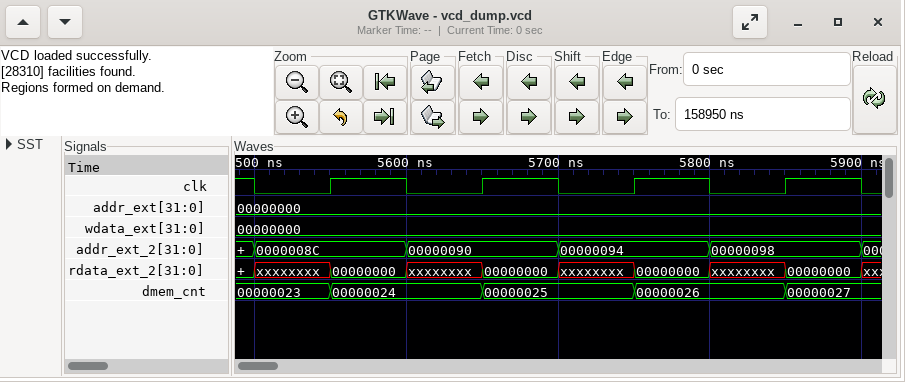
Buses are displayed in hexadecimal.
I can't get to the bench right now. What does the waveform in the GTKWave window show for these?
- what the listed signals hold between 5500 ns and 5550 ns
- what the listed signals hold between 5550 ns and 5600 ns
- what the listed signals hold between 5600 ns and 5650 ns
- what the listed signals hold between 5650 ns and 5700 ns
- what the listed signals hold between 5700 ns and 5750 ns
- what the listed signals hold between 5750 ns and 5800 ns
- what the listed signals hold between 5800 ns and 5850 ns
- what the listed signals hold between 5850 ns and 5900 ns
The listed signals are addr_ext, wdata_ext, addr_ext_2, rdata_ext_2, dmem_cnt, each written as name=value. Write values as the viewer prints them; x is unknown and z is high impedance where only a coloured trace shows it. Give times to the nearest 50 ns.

addr_ext=00000000, wdata_ext=00000000, addr_ext_2=0000008C, rdata_ext_2=xxxxxxxx, dmem_cnt=00000023
addr_ext=00000000, wdata_ext=00000000, addr_ext_2=0000008C, rdata_ext_2=00000000, dmem_cnt=00000024
addr_ext=00000000, wdata_ext=00000000, addr_ext_2=00000090, rdata_ext_2=xxxxxxxx, dmem_cnt=00000024
addr_ext=00000000, wdata_ext=00000000, addr_ext_2=00000090, rdata_ext_2=00000000, dmem_cnt=00000025
addr_ext=00000000, wdata_ext=00000000, addr_ext_2=00000094, rdata_ext_2=xxxxxxxx, dmem_cnt=00000025
addr_ext=00000000, wdata_ext=00000000, addr_ext_2=00000094, rdata_ext_2=00000000, dmem_cnt=00000026
addr_ext=00000000, wdata_ext=00000000, addr_ext_2=00000098, rdata_ext_2=xxxxxxxx, dmem_cnt=00000026
addr_ext=00000000, wdata_ext=00000000, addr_ext_2=00000098, rdata_ext_2=00000000, dmem_cnt=00000027
